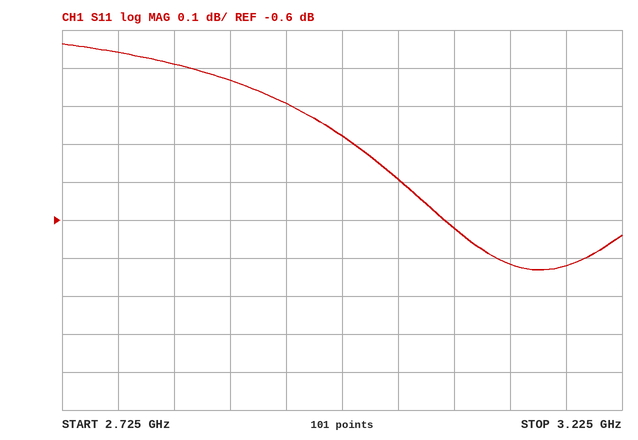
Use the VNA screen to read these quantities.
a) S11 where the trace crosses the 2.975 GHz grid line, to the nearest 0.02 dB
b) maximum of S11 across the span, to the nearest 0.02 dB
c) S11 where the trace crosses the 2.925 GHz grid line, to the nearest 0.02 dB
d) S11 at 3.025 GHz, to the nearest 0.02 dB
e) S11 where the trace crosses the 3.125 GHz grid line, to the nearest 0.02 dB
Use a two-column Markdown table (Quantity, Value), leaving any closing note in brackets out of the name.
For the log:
| Quantity | Value |
|---|---|
| S11 where the trace crosses the 2.975 GHz grid line, to the nearest 0.02 dB | -0.38 dB |
| maximum of S11 across the span, to the nearest 0.02 dB | -0.14 dB |
| S11 where the trace crosses the 2.925 GHz grid line, to the nearest 0.02 dB | -0.30 dB |
| S11 at 3.025 GHz, to the nearest 0.02 dB | -0.50 dB |
| S11 where the trace crosses the 3.125 GHz grid line, to the nearest 0.02 dB | -0.72 dB |
